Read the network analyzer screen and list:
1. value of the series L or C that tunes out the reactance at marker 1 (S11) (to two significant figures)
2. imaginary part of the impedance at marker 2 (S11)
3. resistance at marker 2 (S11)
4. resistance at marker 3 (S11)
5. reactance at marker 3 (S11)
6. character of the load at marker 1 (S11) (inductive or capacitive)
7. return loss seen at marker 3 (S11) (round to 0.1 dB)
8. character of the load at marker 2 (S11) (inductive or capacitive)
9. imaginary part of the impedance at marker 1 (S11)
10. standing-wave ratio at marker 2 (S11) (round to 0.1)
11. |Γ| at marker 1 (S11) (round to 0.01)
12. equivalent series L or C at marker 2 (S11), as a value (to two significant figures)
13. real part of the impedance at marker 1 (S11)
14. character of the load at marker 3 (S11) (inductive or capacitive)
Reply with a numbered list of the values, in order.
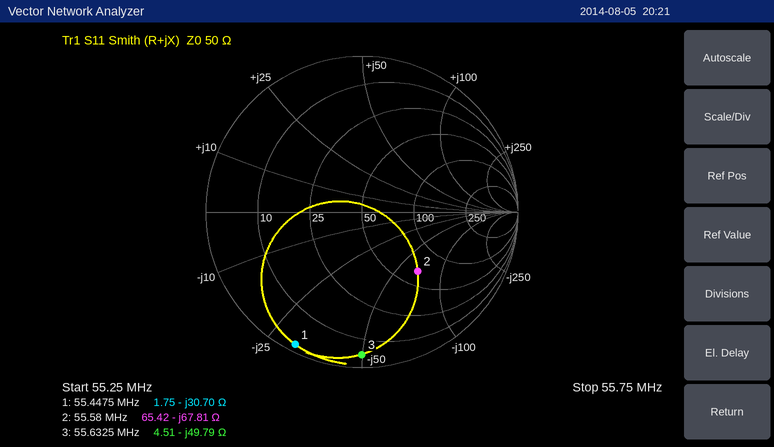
1. 88 nH
2. -67.81 Ω
3. 65.42 Ω
4. 4.51 Ω
5. -49.79 Ω
6. capacitive
7. 0.8 dB
8. capacitive
9. -30.70 Ω
10. 3.2
11. 0.95
12. 42 pF
13. 1.75 Ω
14. capacitive
